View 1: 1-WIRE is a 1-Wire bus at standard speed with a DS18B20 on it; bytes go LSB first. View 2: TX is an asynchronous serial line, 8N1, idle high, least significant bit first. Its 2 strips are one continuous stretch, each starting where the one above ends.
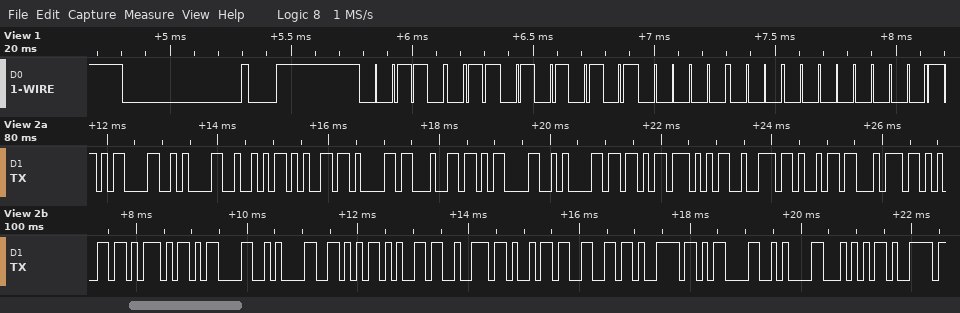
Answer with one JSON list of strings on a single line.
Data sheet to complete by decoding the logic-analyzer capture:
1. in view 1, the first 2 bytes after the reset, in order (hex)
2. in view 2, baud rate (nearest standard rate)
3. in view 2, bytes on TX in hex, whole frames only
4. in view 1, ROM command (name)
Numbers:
["CC AA", "9600 baud", "0D 0A 52 65 61 64 0D 0A 5B 57 72 69 74 65 5D 0D 0A 56 65 72 69 66 79 0D 0A 54 79", "Skip ROM"]
